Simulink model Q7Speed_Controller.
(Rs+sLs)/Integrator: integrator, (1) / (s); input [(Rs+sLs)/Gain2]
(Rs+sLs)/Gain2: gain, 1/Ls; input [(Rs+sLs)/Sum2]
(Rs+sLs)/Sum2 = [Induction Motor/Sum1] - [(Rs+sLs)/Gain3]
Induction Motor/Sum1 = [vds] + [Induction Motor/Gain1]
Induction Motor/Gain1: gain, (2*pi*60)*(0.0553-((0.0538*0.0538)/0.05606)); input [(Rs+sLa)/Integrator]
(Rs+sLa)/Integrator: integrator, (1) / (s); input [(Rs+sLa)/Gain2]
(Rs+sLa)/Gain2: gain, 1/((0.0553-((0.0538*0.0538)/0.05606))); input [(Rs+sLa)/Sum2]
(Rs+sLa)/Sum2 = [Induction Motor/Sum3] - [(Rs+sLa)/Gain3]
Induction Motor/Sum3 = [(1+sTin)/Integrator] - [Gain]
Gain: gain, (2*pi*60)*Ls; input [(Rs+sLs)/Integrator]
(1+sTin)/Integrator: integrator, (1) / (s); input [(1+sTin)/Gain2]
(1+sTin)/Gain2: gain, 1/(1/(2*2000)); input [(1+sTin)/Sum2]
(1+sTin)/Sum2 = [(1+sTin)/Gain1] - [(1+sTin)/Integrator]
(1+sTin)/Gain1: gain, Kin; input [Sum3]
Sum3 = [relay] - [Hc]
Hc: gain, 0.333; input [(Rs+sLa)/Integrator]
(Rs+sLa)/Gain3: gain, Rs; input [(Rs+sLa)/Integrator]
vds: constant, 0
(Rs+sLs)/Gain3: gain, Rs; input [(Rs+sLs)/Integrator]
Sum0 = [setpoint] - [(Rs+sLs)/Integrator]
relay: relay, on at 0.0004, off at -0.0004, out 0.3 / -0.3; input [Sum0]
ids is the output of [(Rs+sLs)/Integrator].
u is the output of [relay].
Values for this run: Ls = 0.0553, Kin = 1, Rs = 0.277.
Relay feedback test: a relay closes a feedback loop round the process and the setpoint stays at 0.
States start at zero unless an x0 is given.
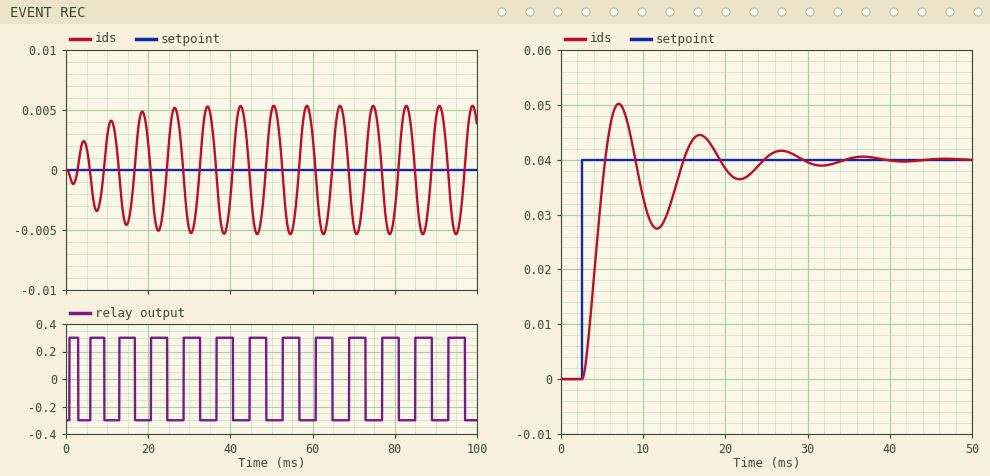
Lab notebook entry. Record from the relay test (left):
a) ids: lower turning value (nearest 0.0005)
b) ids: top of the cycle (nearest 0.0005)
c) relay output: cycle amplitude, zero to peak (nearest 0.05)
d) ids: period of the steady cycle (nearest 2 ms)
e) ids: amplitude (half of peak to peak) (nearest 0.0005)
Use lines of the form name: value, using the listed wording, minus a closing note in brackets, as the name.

ids: lower turning value: -0.0055
ids: top of the cycle: 0.0055
relay output: cycle amplitude, zero to peak: 0.30
ids: period of the steady cycle: 8 ms
ids: amplitude (half of peak to peak): 0.0055
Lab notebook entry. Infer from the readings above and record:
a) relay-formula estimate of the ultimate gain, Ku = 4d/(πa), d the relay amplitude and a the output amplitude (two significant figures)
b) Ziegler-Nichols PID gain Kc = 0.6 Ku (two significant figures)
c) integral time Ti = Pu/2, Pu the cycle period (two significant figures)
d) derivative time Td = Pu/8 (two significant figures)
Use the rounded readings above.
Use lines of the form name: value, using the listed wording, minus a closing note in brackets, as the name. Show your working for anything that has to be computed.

relay-formula estimate of the ultimate gain, Ku = 4d/(πa), d the relay amplitude and a the output amplitude: 4 × 0.3 / (π × 0.0055) = 69
Ziegler-Nichols PID gain Kc = 0.6 Ku: 0.6 × 69 = 41
integral time Ti = Pu/2, Pu the cycle period: 8 / 2 = 4.0 ms
derivative time Td = Pu/8: 8 / 8 = 1.0 ms
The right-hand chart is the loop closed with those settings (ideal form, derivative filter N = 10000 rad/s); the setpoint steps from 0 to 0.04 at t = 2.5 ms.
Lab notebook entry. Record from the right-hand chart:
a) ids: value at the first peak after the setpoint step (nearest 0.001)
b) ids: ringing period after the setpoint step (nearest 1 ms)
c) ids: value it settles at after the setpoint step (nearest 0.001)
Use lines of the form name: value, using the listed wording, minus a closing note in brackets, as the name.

ids: value at the first peak after the setpoint step: 0.050
ids: ringing period after the setpoint step: 10 ms
ids: value it settles at after the setpoint step: 0.040
